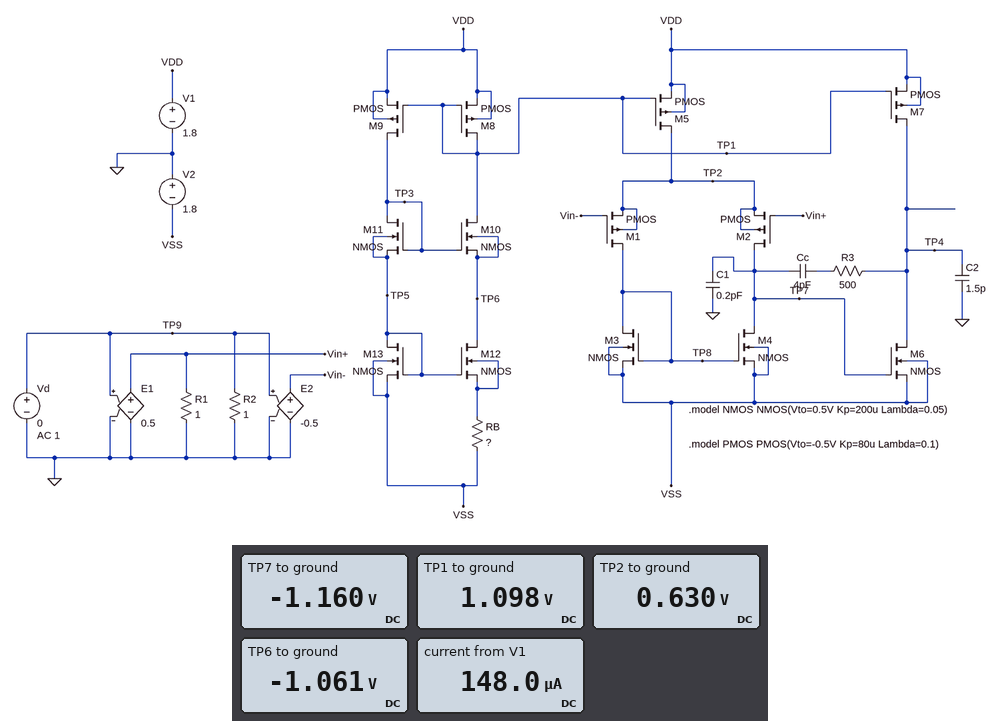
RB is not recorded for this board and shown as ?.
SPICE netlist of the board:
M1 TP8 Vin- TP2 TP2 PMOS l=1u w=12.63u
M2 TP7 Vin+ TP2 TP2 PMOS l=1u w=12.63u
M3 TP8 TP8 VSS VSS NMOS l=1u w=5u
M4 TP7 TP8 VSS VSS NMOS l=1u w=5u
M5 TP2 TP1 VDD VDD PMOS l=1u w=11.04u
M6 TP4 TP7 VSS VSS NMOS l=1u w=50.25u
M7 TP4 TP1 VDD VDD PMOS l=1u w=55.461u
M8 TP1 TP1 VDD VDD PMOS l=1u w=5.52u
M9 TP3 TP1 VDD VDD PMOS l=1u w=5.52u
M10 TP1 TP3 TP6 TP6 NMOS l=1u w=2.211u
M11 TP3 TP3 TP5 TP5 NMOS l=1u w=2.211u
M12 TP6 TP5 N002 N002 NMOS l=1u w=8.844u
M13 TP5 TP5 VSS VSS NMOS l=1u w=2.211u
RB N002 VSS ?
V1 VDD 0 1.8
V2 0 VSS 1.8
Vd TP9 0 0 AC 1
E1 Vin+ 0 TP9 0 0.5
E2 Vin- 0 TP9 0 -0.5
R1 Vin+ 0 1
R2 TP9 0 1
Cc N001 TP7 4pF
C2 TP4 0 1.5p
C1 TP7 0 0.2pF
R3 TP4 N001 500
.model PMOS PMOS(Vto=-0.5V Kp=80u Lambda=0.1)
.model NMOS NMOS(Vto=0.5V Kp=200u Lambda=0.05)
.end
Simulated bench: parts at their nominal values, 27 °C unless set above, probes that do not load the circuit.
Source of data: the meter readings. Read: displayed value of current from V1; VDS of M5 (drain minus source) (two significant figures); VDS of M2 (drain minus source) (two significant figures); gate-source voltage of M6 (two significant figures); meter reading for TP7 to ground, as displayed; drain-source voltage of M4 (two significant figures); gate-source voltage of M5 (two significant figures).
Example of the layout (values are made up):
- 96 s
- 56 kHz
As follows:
- 148.0 µA
- -1.2 V
- -1.8 V
- 640 mV
- -1.160 V
- 640 mV
- -700 mV
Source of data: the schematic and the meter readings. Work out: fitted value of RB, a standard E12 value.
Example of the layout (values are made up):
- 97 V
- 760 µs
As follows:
- 12 kΩ
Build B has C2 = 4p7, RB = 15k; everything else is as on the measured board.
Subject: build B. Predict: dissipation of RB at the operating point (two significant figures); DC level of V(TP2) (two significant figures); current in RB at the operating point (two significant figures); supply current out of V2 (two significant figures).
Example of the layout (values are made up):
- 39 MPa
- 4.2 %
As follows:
- 600 nW
- 610 mV
- 6.3 µA
- 97 µA
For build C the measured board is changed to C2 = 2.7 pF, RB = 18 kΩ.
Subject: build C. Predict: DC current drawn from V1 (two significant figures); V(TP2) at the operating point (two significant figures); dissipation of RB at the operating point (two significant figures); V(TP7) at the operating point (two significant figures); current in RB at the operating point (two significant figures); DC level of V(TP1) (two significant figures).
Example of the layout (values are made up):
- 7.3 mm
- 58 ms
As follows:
- 69 µA
- 590 mV
- 360 nW
- -1.2 V
- 4.5 µA
- 1.2 V
